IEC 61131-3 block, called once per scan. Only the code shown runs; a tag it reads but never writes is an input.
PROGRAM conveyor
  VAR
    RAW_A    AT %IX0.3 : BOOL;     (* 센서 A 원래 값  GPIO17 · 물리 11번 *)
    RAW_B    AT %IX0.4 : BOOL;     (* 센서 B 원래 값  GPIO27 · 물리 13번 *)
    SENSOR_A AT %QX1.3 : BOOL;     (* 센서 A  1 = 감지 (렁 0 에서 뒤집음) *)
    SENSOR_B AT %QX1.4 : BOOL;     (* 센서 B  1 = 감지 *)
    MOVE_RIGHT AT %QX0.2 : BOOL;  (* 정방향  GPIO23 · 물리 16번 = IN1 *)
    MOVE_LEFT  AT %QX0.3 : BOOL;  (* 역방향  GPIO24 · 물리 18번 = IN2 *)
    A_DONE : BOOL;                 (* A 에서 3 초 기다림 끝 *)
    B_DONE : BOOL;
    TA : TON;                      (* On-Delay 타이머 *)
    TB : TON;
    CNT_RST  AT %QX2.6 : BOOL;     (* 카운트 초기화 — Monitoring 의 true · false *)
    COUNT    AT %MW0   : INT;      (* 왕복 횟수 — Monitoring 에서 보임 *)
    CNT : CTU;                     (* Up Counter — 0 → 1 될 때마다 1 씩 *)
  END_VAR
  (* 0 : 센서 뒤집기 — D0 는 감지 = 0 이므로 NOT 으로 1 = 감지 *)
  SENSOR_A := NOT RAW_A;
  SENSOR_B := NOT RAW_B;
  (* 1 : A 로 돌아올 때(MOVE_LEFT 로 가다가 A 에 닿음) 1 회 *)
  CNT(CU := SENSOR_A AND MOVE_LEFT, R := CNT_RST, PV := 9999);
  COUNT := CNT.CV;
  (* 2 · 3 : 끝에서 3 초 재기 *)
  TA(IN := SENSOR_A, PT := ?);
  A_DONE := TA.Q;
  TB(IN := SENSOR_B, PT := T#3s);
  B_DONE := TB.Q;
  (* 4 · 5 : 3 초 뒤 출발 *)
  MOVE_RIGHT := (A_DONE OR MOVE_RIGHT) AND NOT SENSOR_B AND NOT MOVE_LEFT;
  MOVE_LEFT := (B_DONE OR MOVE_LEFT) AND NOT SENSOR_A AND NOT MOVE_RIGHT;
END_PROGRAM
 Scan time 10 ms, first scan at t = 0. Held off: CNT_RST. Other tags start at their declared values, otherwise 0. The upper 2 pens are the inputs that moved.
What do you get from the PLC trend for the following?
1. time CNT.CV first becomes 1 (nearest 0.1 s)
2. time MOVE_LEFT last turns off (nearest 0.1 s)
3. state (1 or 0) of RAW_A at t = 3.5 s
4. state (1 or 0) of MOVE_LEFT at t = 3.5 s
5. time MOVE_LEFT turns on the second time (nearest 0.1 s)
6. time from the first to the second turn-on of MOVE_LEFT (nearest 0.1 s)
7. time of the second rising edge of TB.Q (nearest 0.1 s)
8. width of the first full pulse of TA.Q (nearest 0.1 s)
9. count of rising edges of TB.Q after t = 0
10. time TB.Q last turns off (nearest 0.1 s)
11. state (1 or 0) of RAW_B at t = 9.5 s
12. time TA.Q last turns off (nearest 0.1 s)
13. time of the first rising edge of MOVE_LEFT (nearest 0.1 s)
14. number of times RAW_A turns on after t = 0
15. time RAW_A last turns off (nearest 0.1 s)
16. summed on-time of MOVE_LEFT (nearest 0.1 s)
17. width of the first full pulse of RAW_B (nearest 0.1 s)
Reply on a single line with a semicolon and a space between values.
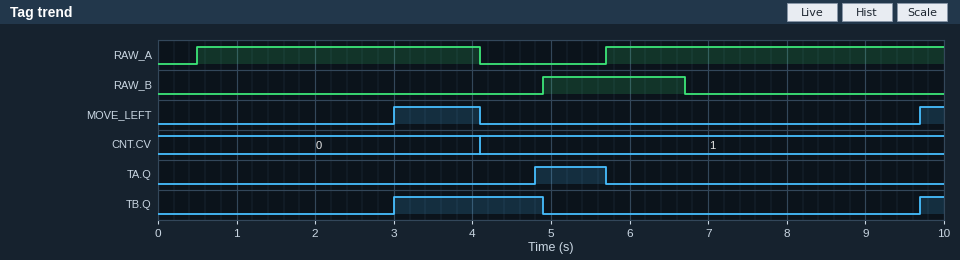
4.1 s; 4.1 s; 1; 1; 9.7 s; 6.7 s; 9.7 s; 0.9 s; 2; 4.9 s; 0; 5.7 s; 3.0 s; 2; 4.1 s; 1.4 s; 1.8 s
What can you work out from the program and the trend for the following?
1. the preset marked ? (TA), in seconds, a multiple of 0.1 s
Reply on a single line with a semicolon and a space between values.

0.7 s
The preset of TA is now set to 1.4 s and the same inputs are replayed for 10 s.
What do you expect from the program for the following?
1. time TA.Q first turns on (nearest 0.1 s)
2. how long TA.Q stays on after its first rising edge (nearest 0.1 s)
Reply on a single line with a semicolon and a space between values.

5.5 s; 0.2 s
